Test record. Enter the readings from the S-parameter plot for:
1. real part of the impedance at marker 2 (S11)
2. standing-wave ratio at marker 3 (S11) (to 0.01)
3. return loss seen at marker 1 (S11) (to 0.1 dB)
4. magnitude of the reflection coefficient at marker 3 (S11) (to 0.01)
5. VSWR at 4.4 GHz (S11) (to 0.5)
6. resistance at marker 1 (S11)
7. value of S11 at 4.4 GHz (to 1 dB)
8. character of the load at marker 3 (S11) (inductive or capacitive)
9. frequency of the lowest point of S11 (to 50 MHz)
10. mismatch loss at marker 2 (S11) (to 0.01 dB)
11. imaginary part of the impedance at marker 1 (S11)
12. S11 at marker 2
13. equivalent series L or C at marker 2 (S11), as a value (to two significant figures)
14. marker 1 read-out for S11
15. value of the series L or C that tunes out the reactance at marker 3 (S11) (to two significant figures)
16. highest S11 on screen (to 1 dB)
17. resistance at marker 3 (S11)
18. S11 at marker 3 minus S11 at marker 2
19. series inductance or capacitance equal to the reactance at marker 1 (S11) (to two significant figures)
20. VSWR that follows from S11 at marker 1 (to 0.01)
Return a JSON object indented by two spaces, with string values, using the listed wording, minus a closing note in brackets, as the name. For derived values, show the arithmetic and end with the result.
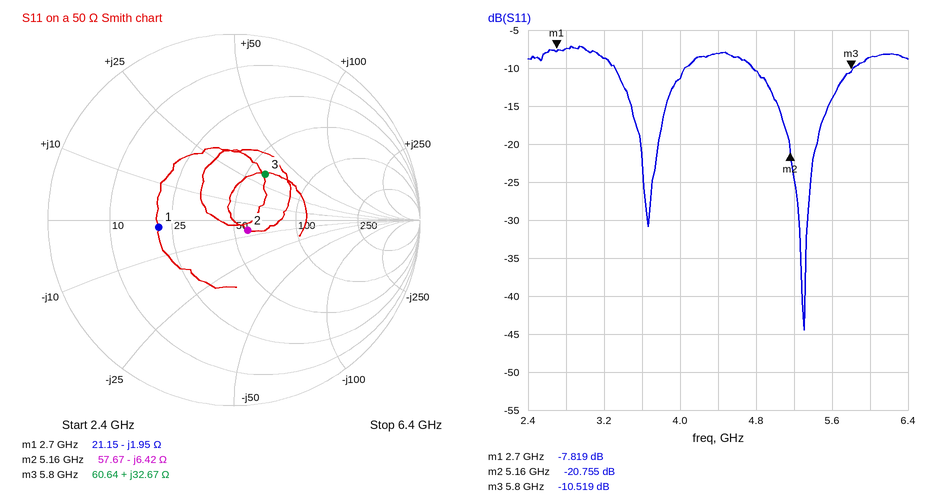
{
  "real part of the impedance at marker 2": "57.67 Ω",
  "standing-wave ratio at marker 3 (S11)": "1.85",
  "return loss seen at marker 1 (S11)": "7.8 dB",
  "magnitude of the reflection coefficient at marker 3 (S11)": "10^(-10.519/20) ≈ 0.30",
  "VSWR at 4.4 GHz (S11)": "|Γ| = 10^(-8/20) = 0.3981; VSWR = (1 + 0.3981)/(1 − 0.3981) ≈ 2.32, so 2.5 to the nearest 0.5",
  "resistance at marker 1": "21.15 Ω",
  "value of S11 at 4.4 GHz": "-8 dB",
  "character of the load at marker 3 (S11)": "inductive",
  "frequency of the lowest point of S11": "5.30 GHz",
  "mismatch loss at marker 2 (S11)": "−10 log10(1 − 10^(-20.755/10)) ≈ 0.04 dB",
  "imaginary part of the impedance at marker 1": "-1.95 Ω",
  "S11 at marker 2": "-20.755 dB",
  "equivalent series L or C at marker 2 (S11), as a value": "C = 1/(2π × 5.16 GHz × 6.42 Ω) ≈ 4.8 pF",
  "marker 1 read-out for S11": "-7.819 dB",
  "value of the series L or C that tunes out the reactance at marker 3 (S11)": "C = 1/(2π × 5.8 GHz × 32.67 Ω) ≈ 840 fF",
  "highest S11 on screen": "-7 dB",
  "resistance at marker 3": "60.64 Ω",
  "S11 at marker 3 minus S11 at marker 2": "-10.519 − (-20.755) = 10.236 dB",
  "series inductance or capacitance equal to the reactance at marker 1 (S11)": "C = 1/(2π × 2.7 GHz × 1.95 Ω) ≈ 30 pF",
  "VSWR that follows from S11 at marker 1": "(1 + 0.4065)/(1 − 0.4065) ≈ 2.37"
}
